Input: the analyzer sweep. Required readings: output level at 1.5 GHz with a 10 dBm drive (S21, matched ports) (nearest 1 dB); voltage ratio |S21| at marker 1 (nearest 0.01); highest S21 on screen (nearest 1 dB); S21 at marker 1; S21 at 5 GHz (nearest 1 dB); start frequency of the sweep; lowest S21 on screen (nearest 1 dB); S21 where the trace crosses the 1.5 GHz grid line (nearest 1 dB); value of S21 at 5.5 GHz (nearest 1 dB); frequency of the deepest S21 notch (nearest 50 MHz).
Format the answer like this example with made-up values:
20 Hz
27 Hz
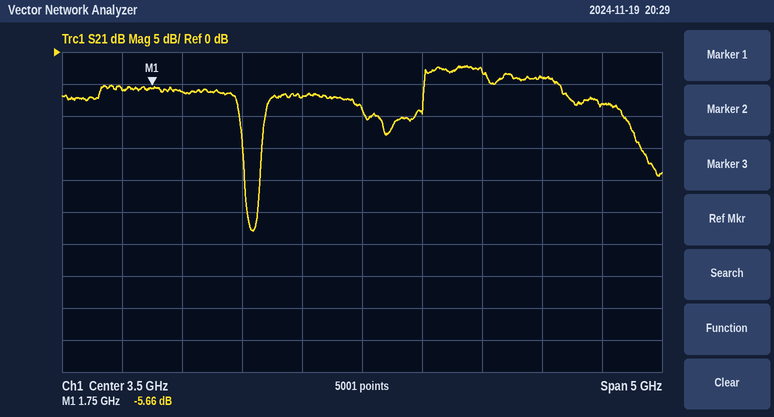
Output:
4 dBm
0.52
-2 dB
-5.66 dB
-4 dB
1 GHz
-28 dB
-6 dB
-8 dB
2.60 GHz
